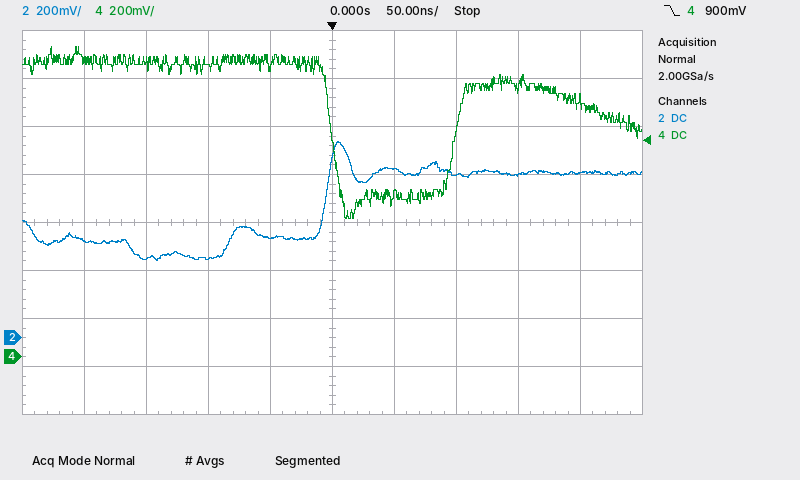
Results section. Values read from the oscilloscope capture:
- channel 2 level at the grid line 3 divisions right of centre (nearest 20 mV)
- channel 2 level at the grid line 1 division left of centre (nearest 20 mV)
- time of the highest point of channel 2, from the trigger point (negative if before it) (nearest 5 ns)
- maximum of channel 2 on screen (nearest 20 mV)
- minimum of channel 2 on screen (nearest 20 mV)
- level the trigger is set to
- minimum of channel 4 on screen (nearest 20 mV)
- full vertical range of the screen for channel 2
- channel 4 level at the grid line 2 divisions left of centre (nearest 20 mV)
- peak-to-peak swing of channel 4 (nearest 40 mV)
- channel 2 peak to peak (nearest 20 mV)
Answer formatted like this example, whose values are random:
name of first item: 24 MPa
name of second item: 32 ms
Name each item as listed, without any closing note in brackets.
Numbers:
channel 2 level at the grid line 3 divisions right of centre: 680 mV
channel 2 level at the grid line 1 division left of centre: 420 mV
time of the highest point of channel 2, from the trigger point (negative if before it): +5 ns
maximum of channel 2 on screen: 820 mV
minimum of channel 2 on screen: 320 mV
level the trigger is set to: 900 mV
minimum of channel 4 on screen: 580 mV
full vertical range of the screen for channel 2: 1.6 V
channel 4 level at the grid line 2 divisions left of centre: 1.20 V
peak-to-peak swing of channel 4: 720 mV
channel 2 peak to peak: 500 mV
